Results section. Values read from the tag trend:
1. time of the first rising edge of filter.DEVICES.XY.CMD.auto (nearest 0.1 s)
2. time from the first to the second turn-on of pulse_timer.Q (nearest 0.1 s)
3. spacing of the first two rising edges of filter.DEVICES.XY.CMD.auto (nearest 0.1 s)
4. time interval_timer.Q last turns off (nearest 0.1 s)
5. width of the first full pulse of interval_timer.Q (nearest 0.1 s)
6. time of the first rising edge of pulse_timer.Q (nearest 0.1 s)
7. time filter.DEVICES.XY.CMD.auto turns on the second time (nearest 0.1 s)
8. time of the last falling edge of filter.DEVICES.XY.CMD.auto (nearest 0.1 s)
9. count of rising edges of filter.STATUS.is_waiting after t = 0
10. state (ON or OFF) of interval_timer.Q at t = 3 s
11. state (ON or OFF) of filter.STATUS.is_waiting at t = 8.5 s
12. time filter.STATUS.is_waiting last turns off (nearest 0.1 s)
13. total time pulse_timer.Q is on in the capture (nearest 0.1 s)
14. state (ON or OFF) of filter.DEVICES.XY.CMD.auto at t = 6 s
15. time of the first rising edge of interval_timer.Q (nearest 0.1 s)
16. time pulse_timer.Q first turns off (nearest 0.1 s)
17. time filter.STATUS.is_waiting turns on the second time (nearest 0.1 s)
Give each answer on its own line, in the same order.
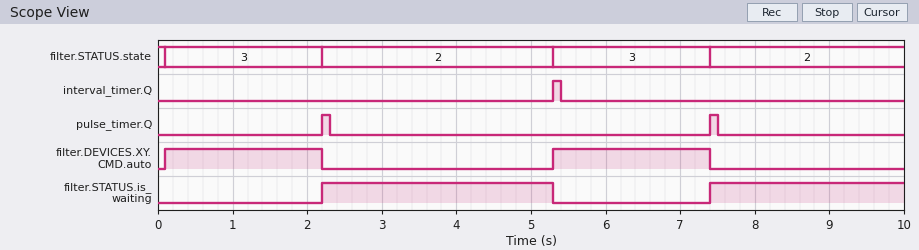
0.1 s
5.2 s
5.2 s
5.4 s
0.1 s
2.2 s
5.3 s
7.4 s
2
OFF
ON
5.3 s
0.2 s
ON
5.3 s
2.3 s
7.4 s
